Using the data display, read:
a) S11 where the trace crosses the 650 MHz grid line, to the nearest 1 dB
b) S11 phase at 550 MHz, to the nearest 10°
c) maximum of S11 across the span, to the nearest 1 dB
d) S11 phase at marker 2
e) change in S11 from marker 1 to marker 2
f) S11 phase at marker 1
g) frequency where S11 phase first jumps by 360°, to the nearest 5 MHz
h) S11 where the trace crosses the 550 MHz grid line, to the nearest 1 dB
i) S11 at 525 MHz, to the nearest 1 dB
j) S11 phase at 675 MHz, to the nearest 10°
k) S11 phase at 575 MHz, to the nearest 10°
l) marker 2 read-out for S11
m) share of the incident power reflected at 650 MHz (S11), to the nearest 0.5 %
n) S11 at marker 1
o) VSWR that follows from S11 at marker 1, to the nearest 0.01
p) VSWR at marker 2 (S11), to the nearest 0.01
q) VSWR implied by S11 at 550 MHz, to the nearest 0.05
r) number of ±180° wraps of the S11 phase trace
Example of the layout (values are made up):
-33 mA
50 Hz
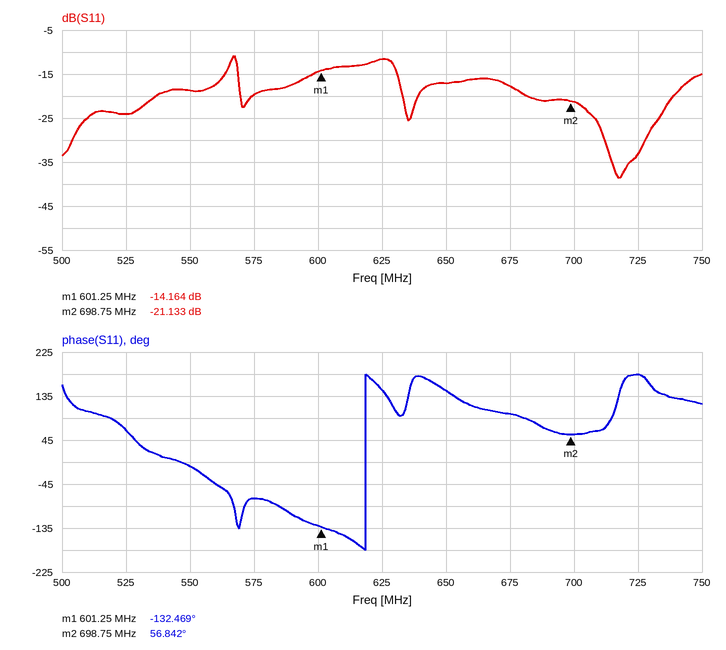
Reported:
-17 dB
-10°
-11 dB
56.842°
-6.969 dB
-132.469°
620 MHz
-19 dB
-24 dB
100°
-70°
-21.133 dB
2.0 %
-14.164 dB
1.49
1.19
1.25
1
